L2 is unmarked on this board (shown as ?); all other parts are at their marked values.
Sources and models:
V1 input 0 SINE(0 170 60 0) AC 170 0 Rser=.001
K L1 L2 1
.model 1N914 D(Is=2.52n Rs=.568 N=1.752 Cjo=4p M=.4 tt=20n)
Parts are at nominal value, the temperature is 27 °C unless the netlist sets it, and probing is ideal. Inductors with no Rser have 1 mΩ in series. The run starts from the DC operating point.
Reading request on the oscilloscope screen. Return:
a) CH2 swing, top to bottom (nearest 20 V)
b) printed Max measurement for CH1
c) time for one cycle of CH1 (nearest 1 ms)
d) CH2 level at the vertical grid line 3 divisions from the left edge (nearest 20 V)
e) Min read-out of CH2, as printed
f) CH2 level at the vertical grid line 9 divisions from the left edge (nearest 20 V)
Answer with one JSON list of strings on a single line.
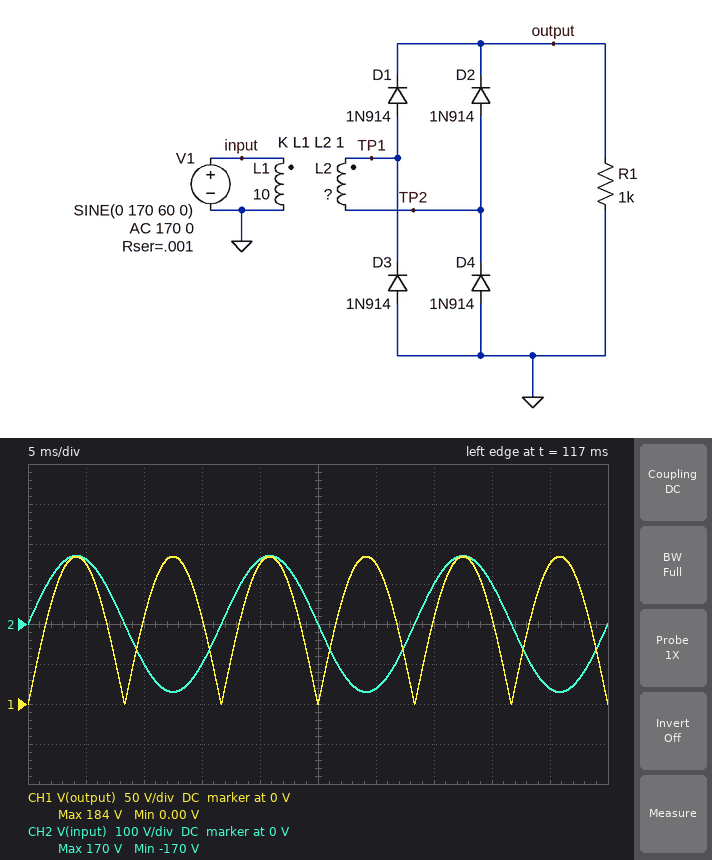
["340 V", "184 V", "8 ms", "-100 V", "-170 V", "-160 V"]
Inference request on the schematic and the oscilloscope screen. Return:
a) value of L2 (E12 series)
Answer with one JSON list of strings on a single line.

["12 H"]
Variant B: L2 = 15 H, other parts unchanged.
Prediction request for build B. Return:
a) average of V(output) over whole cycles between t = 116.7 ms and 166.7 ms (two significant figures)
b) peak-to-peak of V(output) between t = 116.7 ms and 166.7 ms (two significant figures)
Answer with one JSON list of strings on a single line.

["130 V", "210 V"]
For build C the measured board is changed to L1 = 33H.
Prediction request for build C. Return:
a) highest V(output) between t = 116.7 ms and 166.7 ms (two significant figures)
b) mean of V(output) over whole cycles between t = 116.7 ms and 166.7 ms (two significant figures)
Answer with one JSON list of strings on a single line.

["100 V", "64 V"]
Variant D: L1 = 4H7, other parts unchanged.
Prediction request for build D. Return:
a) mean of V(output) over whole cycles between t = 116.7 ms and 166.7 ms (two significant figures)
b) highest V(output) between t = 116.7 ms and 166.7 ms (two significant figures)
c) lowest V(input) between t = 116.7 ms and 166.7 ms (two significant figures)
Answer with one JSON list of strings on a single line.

["170 V", "270 V", "-170 V"]
